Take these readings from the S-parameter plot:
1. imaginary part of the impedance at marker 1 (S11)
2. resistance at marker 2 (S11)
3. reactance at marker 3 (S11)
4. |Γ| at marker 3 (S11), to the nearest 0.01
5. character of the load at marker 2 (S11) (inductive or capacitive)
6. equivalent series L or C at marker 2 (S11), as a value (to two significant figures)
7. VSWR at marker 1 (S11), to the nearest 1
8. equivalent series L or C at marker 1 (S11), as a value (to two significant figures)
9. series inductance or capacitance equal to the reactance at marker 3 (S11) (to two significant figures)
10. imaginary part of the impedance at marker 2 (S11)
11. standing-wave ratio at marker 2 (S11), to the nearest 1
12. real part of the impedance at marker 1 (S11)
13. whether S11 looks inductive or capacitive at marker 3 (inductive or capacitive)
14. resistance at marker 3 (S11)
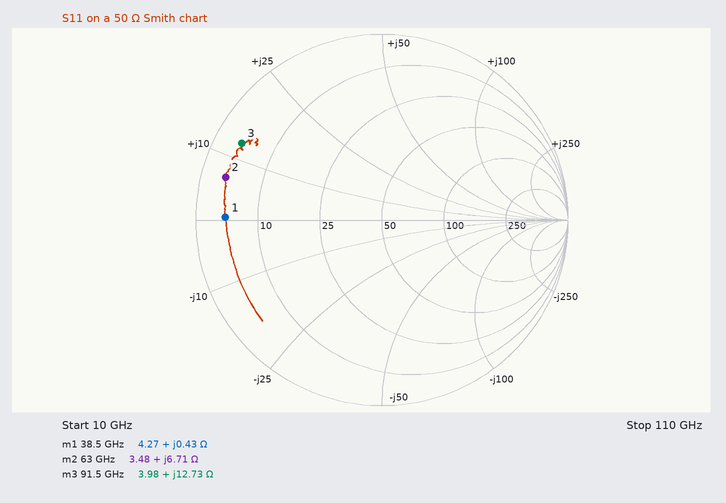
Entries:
+0.43 Ω
3.48 Ω
+12.73 Ω
0.86
inductive
17 pH
12
1.8 pH
22 pH
+6.71 Ω
15
4.27 Ω
inductive
3.98 Ω
